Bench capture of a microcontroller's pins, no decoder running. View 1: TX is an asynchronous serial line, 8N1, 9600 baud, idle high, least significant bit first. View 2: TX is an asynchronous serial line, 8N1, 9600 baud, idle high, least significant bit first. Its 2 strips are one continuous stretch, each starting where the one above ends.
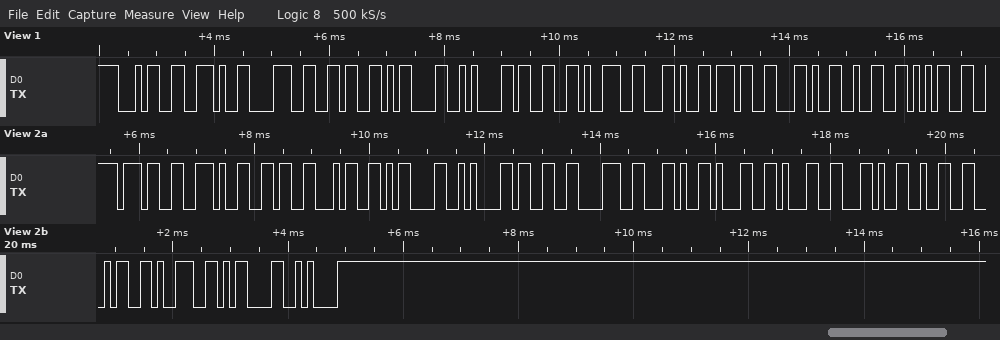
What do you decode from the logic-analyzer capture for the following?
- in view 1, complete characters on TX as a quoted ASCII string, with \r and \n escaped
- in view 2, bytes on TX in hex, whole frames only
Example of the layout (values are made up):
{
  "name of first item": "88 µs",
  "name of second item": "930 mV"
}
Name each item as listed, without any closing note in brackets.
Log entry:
{
  "in view 1, complete characters on TX as a quoted ASCII string, with \\r and \\n escaped": "\"4.86\\r\\n39,7,25\"",
  "in view 2, bytes on TX in hex, whole frames only": "0x37 0x2E 0x36 0x34 0x0D 0x0A 0x33 0x38 0x2C 0x31 0x31 0x2C 0x32 0x34 0x39 0x0D 0x0A"
}
